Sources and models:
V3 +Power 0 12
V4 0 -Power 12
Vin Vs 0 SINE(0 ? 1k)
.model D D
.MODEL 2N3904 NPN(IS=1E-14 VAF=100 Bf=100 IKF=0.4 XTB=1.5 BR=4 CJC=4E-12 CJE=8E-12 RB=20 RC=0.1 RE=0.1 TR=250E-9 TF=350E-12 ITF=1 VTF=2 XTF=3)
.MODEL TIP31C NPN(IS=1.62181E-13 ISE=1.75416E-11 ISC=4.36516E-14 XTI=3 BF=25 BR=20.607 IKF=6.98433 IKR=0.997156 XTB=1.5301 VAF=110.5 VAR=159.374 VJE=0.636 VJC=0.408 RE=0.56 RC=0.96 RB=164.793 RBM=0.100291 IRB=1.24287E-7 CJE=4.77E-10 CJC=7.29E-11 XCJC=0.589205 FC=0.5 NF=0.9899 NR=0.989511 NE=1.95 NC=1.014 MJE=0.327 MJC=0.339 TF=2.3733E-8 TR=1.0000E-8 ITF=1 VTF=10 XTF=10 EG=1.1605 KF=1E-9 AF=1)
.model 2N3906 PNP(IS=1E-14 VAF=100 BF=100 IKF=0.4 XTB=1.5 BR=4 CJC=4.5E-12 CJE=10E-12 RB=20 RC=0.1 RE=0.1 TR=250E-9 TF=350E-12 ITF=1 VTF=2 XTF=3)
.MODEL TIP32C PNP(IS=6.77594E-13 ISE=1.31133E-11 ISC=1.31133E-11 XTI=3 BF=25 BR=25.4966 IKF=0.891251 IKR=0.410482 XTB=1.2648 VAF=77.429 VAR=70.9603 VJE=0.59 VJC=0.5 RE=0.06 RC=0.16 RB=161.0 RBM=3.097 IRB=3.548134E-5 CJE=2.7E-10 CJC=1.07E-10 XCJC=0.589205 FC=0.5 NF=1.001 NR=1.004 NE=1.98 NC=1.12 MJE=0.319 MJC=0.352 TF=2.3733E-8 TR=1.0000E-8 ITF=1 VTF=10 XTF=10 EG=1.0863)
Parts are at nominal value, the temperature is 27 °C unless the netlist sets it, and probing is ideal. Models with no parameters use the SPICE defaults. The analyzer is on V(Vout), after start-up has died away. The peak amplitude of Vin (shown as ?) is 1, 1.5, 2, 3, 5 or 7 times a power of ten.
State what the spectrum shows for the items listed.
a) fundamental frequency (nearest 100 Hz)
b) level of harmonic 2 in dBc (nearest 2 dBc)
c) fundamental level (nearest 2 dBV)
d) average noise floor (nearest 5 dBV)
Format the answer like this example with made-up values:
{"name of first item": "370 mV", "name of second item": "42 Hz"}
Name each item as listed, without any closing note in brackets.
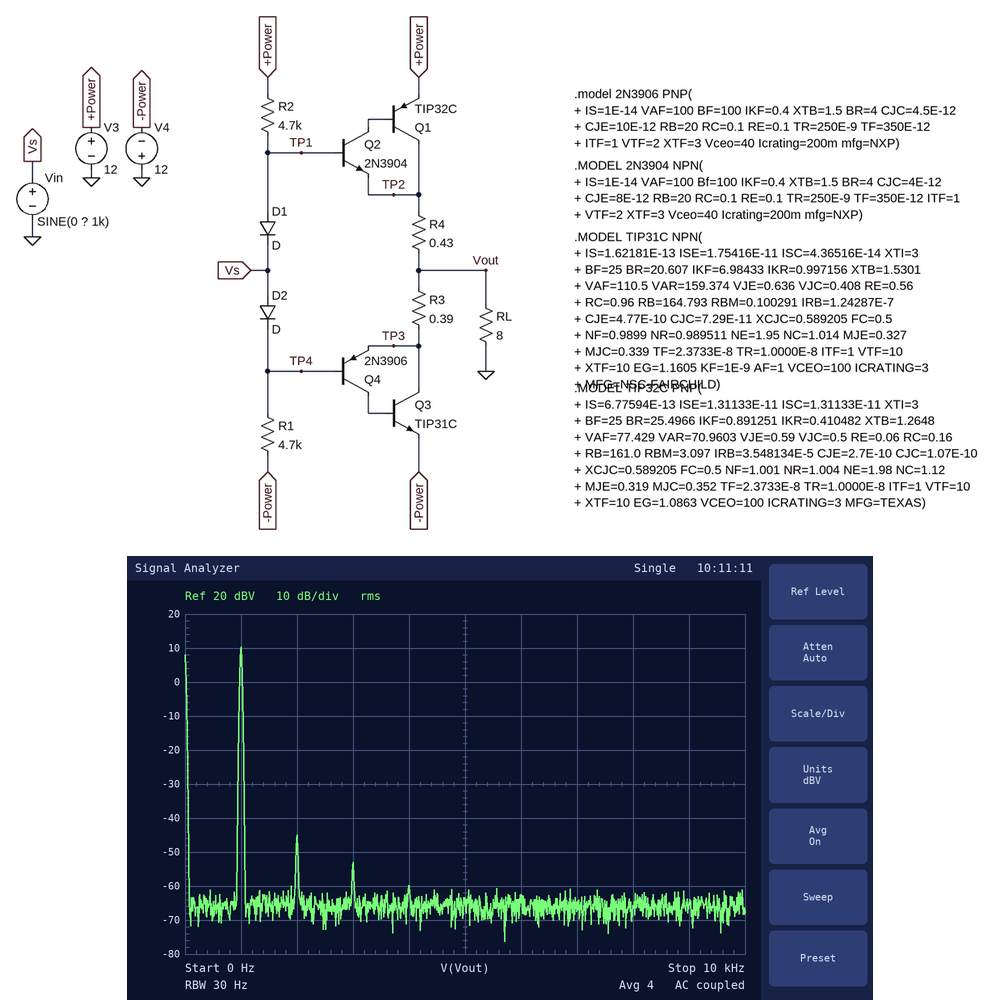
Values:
{"fundamental frequency": "1.0 kHz", "level of harmonic 2 in dBc": "-56 dBc", "fundamental level": "10 dBV", "average noise floor": "-65 dBV"}
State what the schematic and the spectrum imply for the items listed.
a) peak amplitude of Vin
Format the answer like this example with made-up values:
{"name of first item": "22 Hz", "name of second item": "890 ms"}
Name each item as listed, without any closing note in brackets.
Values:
{"peak amplitude of Vin": "5 V"}
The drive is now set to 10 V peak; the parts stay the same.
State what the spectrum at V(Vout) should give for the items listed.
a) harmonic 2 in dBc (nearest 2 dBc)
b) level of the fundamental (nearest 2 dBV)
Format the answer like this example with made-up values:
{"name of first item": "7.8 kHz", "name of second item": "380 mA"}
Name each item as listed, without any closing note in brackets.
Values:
{"harmonic 2 in dBc": "-30 dBc", "level of the fundamental": "16 dBV"}
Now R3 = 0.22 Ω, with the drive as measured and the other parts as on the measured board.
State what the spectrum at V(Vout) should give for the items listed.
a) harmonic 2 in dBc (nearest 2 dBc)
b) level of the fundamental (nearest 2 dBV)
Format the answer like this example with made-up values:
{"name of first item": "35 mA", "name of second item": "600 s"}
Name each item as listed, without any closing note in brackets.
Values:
{"harmonic 2 in dBc": "-44 dBc", "level of the fundamental": "10 dBV"}
